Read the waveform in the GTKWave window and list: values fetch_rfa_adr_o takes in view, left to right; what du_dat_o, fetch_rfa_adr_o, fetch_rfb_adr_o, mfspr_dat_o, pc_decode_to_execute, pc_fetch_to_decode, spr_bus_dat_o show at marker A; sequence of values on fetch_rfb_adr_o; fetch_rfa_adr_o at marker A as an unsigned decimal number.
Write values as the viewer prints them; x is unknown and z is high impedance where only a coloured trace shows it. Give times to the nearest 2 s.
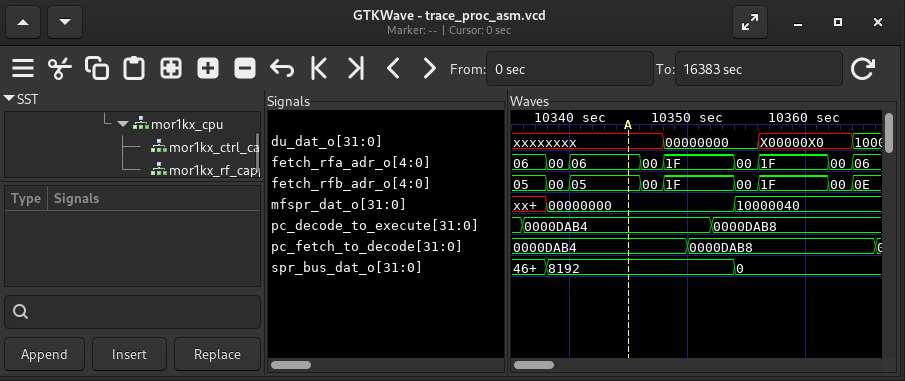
06, 00, 06, 00, 1F, 00, 1F, 00, 06
du_dat_o=xxxxxxxx, fetch_rfa_adr_o=06, fetch_rfb_adr_o=05, mfspr_dat_o=00000000, pc_decode_to_execute=0000DAB4, pc_fetch_to_decode=0000DAB4, spr_bus_dat_o=8192
05, 00, 05, 00, 1F, 00, 1F, 00, 0E
6
